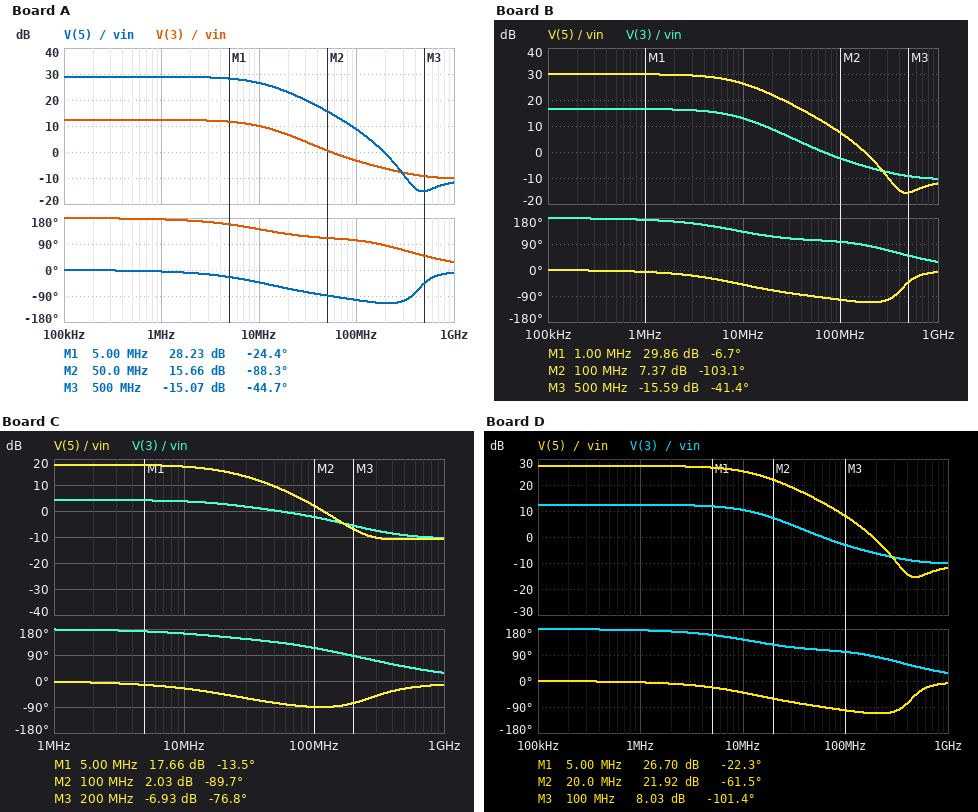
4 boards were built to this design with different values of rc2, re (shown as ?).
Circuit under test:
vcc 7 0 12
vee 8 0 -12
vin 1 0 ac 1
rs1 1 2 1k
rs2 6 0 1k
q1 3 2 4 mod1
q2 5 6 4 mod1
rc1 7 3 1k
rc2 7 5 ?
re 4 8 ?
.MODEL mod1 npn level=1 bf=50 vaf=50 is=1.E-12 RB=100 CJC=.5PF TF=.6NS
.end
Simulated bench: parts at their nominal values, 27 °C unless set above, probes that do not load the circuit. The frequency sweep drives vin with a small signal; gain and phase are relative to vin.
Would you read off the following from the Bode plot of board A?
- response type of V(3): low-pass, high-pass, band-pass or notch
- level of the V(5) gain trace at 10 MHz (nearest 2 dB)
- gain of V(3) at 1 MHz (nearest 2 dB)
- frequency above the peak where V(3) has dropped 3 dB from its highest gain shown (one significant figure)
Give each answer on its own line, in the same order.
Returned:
low-pass
26 dB
12 dB
10 MHz
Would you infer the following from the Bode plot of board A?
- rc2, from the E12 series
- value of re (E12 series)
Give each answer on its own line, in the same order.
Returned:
6.8 kΩ
22 kΩ
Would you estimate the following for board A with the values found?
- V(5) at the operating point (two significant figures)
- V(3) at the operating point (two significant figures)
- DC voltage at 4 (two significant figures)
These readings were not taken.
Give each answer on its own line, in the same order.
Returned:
10 V
12 V
-500 mV
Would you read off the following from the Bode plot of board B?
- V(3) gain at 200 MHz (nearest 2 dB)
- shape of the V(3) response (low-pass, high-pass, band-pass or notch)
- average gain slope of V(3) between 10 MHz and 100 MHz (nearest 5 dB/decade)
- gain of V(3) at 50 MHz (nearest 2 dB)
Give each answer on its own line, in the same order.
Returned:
-6 dB
low-pass
-15 dB/decade
2 dB
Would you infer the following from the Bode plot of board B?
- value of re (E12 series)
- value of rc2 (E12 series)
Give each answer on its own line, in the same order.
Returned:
12 kΩ
4.7 kΩ
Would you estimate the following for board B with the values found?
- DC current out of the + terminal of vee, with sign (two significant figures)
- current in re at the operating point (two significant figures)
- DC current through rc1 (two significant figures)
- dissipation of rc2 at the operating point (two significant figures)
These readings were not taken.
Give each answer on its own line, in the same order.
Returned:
-960 µA
960 µA
480 µA
1.0 mW
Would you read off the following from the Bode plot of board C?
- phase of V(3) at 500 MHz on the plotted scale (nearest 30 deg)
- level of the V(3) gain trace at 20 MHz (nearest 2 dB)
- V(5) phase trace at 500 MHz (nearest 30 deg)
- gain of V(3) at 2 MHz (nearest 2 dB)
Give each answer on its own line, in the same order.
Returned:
60 deg
2 dB
-30 deg
4 dB
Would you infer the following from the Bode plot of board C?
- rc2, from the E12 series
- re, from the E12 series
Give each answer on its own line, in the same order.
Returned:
12 kΩ
4.7 kΩ
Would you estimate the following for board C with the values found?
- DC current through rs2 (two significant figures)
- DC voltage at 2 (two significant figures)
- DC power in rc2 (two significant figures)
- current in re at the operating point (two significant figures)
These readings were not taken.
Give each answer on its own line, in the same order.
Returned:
24 µA
-22 mV
13 mW
2.4 mA
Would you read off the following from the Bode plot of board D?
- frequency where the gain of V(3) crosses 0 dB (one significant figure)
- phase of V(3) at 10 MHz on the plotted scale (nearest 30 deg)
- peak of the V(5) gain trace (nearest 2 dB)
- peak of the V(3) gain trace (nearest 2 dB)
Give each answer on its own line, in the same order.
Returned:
60 MHz
150 deg
28 dB
12 dB
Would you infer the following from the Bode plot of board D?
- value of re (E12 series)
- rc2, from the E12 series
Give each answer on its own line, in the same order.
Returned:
22 kΩ
5.6 kΩ
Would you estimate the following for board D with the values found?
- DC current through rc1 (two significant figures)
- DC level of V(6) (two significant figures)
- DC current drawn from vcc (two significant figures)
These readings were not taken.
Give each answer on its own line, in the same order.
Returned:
260 µA
-4.2 mV
510 µA
